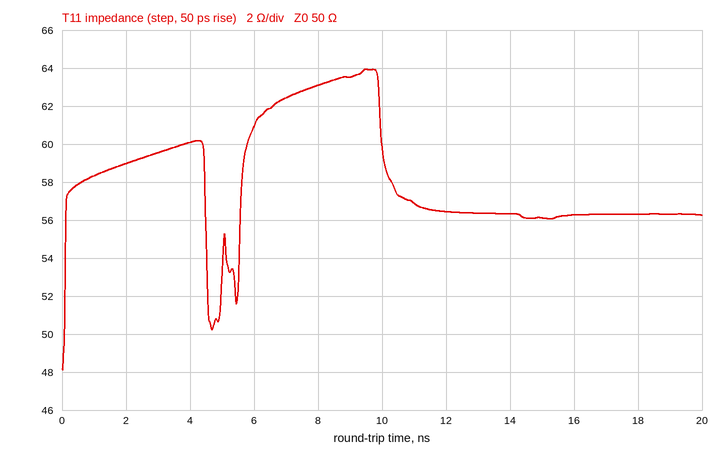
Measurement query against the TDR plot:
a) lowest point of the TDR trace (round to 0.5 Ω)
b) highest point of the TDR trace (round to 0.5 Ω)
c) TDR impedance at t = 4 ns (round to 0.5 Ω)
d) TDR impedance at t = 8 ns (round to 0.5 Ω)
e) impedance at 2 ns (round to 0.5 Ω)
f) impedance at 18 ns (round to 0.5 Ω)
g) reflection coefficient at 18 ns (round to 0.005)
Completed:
48.0 Ω
64.0 Ω
60.0 Ω
63.0 Ω
59.0 Ω
56.5 Ω
+0.060
